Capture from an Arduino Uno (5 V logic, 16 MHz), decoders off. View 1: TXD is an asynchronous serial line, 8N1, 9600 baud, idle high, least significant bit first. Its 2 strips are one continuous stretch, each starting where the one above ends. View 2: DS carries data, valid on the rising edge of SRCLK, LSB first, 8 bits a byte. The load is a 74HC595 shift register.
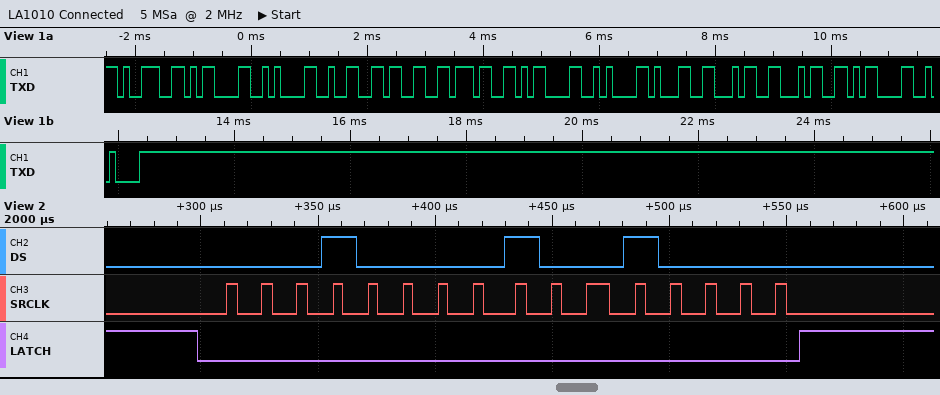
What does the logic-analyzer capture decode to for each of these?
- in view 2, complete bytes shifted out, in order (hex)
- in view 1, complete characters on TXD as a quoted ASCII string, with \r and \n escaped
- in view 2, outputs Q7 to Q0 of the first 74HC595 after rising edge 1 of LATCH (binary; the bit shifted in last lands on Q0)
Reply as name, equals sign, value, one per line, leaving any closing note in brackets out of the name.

in view 2, complete bytes shifted out, in order = 0x08 0x09
in view 1, complete characters on TXD as a quoted ASCII string, with \r and \n escaped = "9\r\n237\r\n144\r\n"
in view 2, outputs Q7 to Q0 of the first 74HC595 after rising edge 1 of LATCH = 10010000
